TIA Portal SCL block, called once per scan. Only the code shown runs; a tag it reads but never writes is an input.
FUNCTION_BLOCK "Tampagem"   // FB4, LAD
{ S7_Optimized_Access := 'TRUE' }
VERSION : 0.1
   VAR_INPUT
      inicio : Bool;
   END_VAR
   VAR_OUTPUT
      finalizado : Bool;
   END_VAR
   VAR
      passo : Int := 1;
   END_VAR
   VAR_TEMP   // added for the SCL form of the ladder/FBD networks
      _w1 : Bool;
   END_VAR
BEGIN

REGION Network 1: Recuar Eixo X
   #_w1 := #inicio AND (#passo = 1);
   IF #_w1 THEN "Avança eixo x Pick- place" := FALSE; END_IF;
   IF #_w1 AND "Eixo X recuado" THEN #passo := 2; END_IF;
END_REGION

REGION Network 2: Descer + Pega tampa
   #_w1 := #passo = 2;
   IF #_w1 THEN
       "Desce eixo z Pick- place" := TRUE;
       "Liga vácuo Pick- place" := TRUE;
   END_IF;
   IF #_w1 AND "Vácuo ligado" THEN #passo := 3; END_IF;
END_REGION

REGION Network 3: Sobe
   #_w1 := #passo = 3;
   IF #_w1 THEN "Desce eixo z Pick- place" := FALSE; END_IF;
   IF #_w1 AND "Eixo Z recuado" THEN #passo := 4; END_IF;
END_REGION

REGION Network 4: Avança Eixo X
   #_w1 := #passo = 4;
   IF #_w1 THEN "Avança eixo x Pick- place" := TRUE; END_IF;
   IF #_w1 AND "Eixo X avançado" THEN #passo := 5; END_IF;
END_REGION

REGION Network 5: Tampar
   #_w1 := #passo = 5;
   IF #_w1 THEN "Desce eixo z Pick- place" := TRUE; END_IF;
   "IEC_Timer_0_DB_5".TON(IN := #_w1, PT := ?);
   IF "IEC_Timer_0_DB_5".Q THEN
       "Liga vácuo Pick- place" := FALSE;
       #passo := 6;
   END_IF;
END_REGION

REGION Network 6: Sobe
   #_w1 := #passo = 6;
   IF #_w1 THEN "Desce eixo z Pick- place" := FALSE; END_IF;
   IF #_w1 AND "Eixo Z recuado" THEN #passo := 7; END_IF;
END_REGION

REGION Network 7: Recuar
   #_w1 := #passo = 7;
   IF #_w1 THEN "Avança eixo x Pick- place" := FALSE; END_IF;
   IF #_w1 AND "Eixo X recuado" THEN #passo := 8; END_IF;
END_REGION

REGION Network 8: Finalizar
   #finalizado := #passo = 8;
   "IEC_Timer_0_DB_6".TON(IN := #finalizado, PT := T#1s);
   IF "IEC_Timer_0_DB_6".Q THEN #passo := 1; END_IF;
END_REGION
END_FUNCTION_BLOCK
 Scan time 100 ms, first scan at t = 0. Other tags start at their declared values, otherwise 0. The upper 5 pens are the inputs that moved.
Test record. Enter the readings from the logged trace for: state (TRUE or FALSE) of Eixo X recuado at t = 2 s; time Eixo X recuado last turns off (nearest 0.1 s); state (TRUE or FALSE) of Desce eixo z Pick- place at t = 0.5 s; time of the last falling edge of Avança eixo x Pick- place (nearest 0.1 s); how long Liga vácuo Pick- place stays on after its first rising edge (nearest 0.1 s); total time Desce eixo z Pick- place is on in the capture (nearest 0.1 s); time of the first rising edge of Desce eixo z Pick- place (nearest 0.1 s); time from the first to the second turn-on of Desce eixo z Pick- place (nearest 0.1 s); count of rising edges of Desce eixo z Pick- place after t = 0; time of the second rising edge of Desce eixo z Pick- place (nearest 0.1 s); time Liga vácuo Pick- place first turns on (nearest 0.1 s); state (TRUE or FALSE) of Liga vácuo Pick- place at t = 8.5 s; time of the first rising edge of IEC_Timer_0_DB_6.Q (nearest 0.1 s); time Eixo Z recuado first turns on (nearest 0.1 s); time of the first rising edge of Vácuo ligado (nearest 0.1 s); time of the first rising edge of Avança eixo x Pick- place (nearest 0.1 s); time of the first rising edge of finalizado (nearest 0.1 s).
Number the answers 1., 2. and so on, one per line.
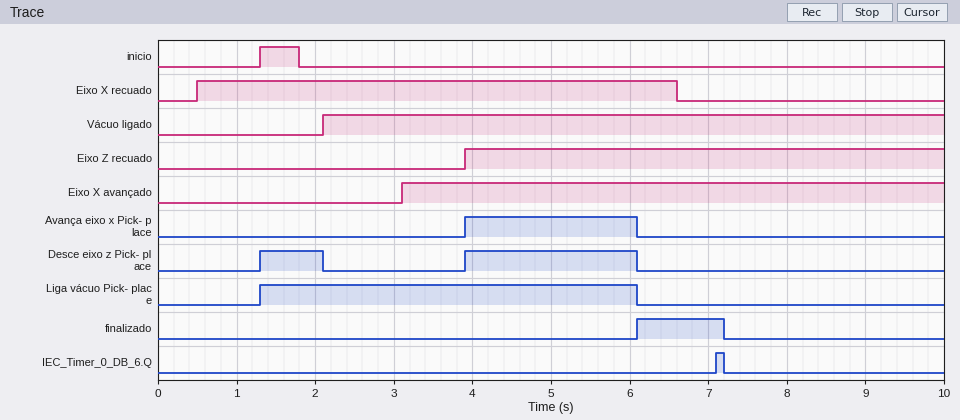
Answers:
1. TRUE
2. 6.6 s
3. FALSE
4. 6.1 s
5. 4.8 s
6. 3.0 s
7. 1.3 s
8. 2.6 s
9. 2
10. 3.9 s
11. 1.3 s
12. FALSE
13. 7.1 s
14. 3.9 s
15. 2.1 s
16. 3.9 s
17. 6.1 s
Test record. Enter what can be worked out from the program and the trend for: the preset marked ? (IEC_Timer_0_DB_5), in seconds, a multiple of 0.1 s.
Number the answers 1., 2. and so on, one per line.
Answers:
1. 2.2 s
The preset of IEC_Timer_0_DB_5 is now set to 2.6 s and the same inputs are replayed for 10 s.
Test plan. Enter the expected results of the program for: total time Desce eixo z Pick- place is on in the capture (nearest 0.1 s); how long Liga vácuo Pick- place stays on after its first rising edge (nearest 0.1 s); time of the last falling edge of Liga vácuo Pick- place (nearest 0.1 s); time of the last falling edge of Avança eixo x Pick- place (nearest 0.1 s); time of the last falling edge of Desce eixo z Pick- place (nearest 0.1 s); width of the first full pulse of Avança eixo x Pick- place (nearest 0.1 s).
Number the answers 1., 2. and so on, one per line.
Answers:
1. 3.4 s
2. 5.2 s
3. 6.5 s
4. 6.5 s
5. 6.5 s
6. 2.6 s
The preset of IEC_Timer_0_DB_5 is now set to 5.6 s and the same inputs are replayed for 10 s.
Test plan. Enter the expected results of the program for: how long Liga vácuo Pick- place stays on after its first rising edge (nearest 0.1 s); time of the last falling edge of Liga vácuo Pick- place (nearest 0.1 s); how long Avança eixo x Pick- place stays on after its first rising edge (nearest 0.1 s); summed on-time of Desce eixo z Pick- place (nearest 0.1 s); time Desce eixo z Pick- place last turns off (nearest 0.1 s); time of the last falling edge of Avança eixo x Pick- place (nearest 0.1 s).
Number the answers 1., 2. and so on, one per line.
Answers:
1. 8.2 s
2. 9.5 s
3. 5.6 s
4. 6.4 s
5. 9.5 s
6. 9.5 s
